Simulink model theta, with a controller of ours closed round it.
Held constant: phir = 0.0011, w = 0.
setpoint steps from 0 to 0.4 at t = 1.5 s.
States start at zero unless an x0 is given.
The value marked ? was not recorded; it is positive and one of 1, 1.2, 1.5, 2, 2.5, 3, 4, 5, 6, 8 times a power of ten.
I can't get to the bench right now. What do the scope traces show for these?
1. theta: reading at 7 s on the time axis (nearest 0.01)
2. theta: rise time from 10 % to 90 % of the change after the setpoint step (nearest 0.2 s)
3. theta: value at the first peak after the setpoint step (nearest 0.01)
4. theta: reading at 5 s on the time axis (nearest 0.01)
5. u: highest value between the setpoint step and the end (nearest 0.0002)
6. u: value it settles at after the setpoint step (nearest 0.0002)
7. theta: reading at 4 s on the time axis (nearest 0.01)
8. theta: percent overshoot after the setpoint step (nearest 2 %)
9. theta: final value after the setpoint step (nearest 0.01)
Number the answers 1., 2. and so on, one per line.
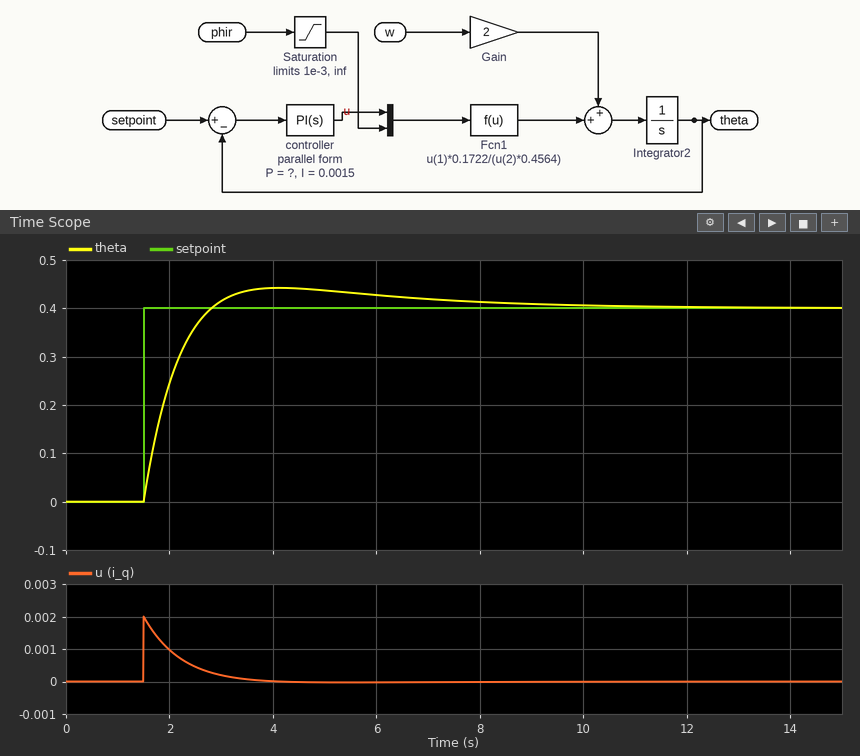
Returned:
1. 0.42
2. 1.0 s
3. 0.44
4. 0.44
5. 0.0020
6. 0.0000
7. 0.44
8. 10 %
9. 0.40
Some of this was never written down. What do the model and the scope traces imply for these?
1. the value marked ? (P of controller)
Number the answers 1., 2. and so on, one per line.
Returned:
1. 0.005
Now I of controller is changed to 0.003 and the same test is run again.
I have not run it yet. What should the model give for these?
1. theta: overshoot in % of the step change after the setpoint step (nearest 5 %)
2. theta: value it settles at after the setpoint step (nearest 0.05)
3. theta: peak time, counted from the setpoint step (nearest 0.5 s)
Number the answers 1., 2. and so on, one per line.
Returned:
1. 15 %
2. 0.40
3. 2.0 s
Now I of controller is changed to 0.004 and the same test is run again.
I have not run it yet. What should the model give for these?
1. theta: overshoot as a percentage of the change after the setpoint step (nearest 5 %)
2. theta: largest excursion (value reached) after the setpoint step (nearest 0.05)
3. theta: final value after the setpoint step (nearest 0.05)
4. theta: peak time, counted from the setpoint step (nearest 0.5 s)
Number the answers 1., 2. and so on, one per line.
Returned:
1. 20 %
2. 0.50
3. 0.40
4. 2.0 s
